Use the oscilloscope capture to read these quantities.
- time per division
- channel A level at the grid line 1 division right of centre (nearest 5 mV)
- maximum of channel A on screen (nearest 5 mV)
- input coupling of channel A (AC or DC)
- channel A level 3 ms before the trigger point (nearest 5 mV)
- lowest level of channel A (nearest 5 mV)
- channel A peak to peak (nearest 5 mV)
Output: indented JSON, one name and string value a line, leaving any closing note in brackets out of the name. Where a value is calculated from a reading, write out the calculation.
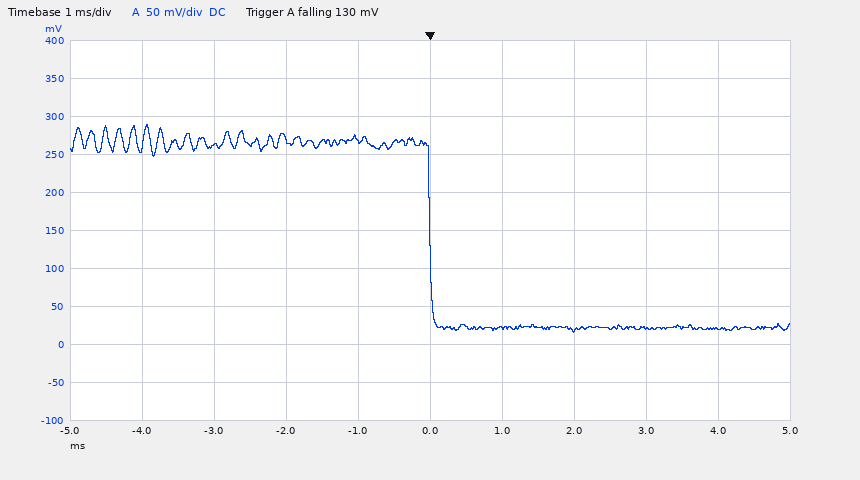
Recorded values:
{
  "time per division": "1 ms",
  "channel A level at the grid line 1 division right of centre": "20 mV",
  "maximum of channel A on screen": "290 mV",
  "input coupling of channel A": "DC",
  "channel A level 3 ms before the trigger point": "260 mV",
  "lowest level of channel A": "15 mV",
  "channel A peak to peak": "290 mV − (15 mV) = 275 mV"
}
